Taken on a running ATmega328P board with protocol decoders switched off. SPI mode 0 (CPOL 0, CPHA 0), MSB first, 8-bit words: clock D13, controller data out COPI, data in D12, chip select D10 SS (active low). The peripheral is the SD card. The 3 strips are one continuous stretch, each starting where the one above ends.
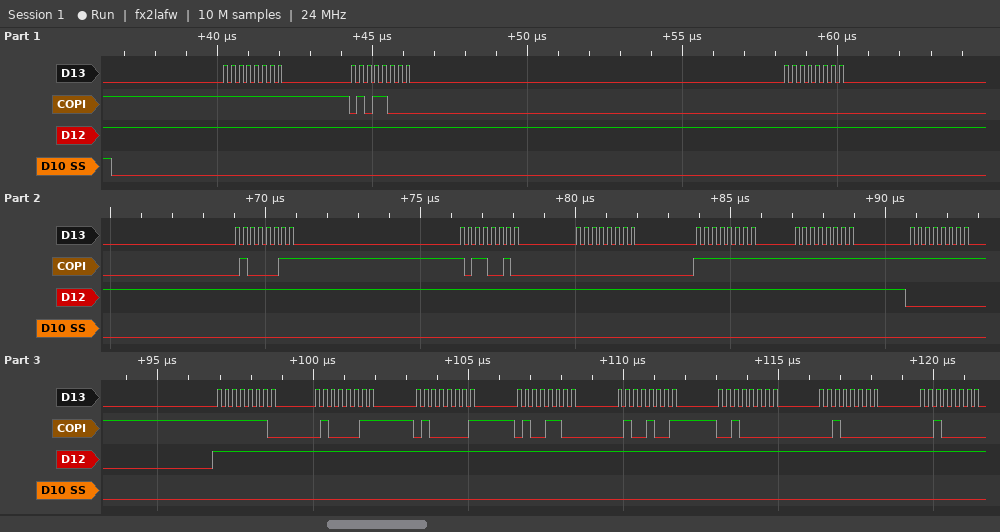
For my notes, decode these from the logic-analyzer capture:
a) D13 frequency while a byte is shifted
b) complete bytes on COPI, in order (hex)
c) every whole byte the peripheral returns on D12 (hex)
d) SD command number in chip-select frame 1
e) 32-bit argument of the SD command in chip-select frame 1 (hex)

4 MHz
FF 58 00 43 B2 00 FF FF FF FE 43 41 4C 49 20 20 20
FF FF FF FF FF FF FF FF 00 FF FF FF FF FF FF FF FF
CMD24
0x0043B200
